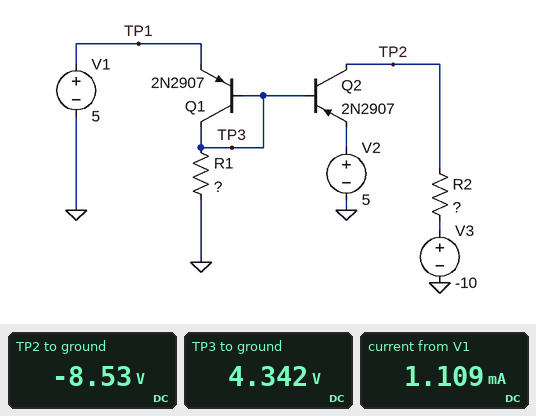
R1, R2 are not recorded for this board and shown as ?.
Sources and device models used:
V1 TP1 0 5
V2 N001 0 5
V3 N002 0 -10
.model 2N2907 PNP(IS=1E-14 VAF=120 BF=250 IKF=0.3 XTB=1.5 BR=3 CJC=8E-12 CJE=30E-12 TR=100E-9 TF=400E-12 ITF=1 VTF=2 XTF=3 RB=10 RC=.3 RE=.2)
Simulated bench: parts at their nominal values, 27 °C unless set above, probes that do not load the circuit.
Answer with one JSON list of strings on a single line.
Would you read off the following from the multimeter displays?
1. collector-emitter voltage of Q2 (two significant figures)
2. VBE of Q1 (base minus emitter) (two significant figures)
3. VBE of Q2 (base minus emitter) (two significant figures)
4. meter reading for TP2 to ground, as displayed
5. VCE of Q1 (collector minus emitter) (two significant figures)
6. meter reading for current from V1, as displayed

["-14 V", "-660 mV", "-660 mV", "-8.53 V", "-660 mV", "1.109 mA"]
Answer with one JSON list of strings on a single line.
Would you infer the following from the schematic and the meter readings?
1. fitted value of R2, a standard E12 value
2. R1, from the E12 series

["1.2 kΩ", "3.9 kΩ"]
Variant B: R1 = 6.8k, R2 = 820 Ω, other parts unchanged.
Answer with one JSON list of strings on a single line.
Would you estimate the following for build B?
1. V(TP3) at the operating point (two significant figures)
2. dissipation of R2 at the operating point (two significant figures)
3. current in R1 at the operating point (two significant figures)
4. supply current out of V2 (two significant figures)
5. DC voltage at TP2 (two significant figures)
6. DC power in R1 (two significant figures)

["4.4 V", "410 µW", "640 µA", "710 µA", "-9.4 V", "2.8 mW"]
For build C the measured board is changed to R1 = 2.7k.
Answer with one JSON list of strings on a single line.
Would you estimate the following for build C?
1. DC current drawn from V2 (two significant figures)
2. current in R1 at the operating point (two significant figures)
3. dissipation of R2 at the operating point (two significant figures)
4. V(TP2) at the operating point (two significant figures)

["1.8 mA", "1.6 mA", "3.7 mW", "-7.9 V"]
